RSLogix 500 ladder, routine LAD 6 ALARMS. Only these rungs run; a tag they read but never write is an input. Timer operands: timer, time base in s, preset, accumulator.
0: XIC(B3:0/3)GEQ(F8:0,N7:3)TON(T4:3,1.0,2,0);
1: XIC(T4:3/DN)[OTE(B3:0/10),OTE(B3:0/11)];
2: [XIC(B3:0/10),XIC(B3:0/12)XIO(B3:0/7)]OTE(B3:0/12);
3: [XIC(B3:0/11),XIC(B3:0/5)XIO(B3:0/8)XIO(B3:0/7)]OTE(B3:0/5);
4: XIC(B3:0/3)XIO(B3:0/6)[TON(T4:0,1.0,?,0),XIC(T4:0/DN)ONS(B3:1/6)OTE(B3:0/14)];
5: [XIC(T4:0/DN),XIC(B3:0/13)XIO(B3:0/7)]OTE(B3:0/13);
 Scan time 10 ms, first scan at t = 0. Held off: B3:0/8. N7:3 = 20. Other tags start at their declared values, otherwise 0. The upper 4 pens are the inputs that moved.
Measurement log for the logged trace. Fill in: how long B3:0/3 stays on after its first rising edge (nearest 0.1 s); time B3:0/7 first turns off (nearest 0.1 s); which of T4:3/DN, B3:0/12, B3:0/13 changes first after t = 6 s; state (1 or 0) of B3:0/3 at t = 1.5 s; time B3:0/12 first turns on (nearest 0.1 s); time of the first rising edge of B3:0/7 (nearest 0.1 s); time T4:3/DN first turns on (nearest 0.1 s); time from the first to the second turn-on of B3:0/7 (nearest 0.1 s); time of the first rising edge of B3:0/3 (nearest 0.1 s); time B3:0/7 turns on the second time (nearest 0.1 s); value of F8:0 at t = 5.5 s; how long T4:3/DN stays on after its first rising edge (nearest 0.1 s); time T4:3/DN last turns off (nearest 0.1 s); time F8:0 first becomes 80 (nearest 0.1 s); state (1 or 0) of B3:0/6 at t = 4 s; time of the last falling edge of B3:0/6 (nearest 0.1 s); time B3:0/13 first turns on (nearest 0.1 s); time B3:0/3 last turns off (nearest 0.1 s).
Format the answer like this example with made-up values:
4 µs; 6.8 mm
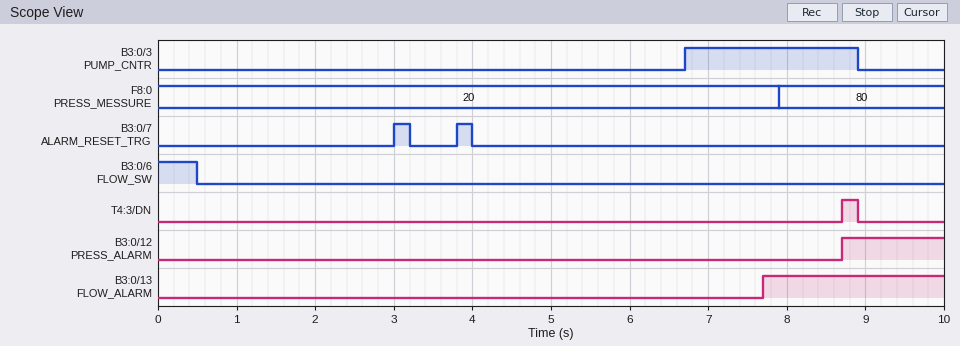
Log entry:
2.2 s; 3.2 s; B3:0/13; 0; 8.7 s; 3.0 s; 8.7 s; 0.8 s; 6.7 s; 3.8 s; 20; 0.2 s; 8.9 s; 7.9 s; 0; 0.5 s; 7.7 s; 8.9 s
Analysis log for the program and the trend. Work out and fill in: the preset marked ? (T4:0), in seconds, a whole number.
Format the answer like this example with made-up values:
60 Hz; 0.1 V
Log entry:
1 s
